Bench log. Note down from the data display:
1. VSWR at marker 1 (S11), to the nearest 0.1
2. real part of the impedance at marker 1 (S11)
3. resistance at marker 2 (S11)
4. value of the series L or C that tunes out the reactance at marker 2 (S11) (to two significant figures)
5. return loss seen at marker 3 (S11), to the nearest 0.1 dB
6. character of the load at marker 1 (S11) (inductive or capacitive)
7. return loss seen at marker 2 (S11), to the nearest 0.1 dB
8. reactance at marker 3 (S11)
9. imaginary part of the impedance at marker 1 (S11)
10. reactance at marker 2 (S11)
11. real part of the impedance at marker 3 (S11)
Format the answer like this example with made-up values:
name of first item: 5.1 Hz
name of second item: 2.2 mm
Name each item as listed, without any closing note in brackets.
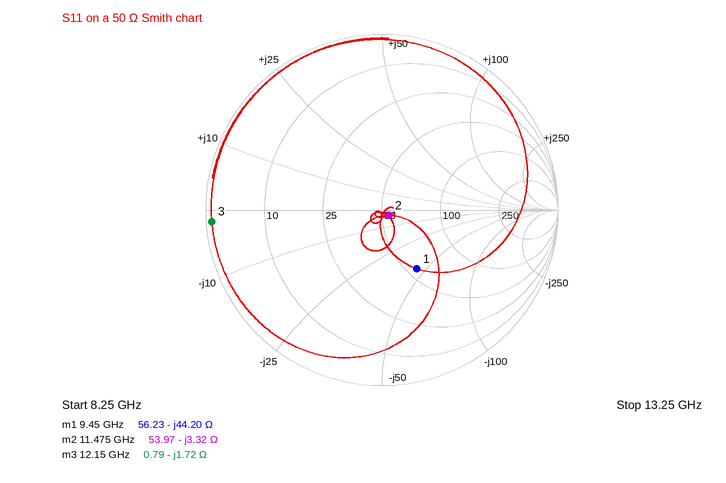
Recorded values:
VSWR at marker 1 (S11), to the nearest 0.1: 2.3
real part of the impedance at marker 1: 56.23 Ω
resistance at marker 2: 53.97 Ω
value of the series L or C that tunes out the reactance at marker 2 (S11): 46 pH
return loss seen at marker 3 (S11), to the nearest 0.1 dB: 0.3 dB
character of the load at marker 1 (S11): capacitive
return loss seen at marker 2 (S11), to the nearest 0.1 dB: 26.1 dB
reactance at marker 3: -1.72 Ω
imaginary part of the impedance at marker 1: -44.20 Ω
reactance at marker 2: -3.32 Ω
real part of the impedance at marker 3: 0.79 Ω
